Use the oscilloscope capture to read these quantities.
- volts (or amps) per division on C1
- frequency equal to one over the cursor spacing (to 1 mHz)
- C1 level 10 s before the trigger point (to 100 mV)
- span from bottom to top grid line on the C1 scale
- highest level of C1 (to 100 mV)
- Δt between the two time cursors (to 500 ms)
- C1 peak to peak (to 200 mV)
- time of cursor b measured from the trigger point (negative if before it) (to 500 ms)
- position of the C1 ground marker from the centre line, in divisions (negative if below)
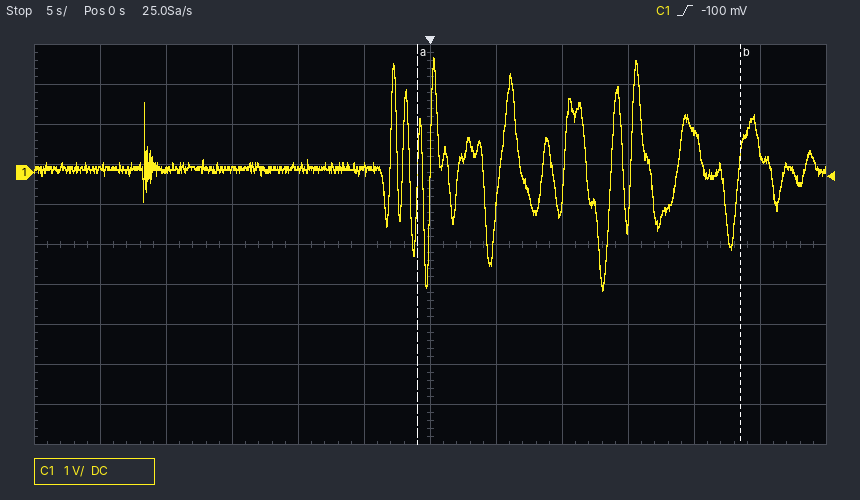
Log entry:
1 V
41 mHz
100 mV
10 V
2.9 V
24.5 s
5.8 V
+23.5 s
+1.8 div
